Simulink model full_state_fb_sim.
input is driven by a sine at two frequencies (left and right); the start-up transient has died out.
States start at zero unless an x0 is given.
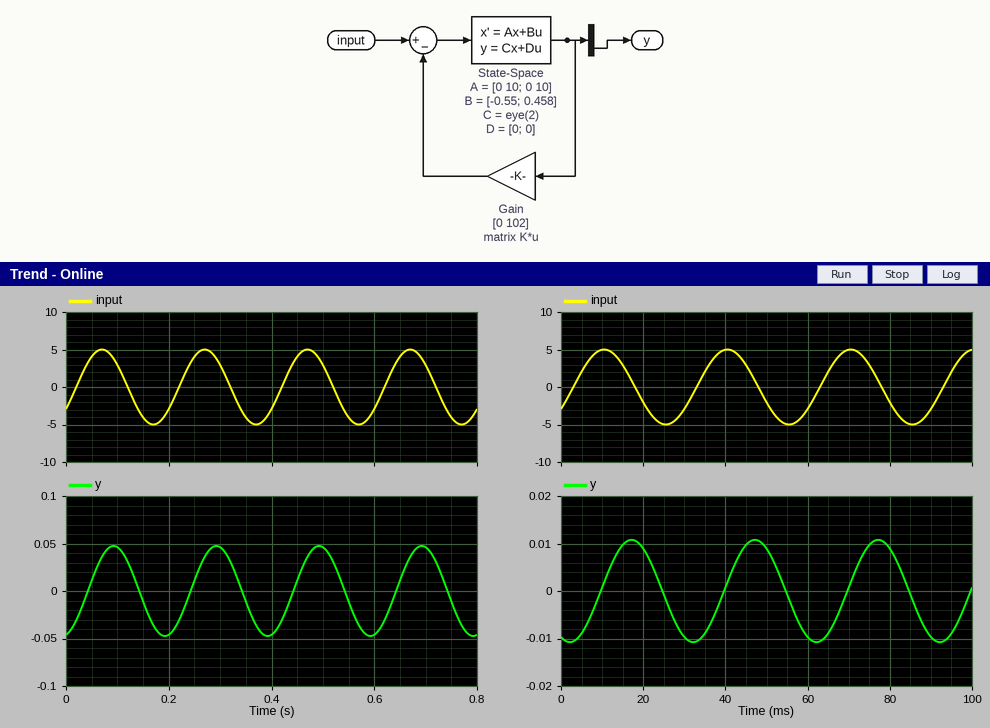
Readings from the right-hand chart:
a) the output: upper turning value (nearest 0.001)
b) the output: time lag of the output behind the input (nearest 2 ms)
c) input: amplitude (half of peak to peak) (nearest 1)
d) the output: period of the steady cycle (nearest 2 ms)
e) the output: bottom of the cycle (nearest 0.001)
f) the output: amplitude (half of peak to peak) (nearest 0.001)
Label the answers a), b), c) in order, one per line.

a) 0.011
b) 6 ms
c) 5
d) 30 ms
e) -0.011
f) 0.011
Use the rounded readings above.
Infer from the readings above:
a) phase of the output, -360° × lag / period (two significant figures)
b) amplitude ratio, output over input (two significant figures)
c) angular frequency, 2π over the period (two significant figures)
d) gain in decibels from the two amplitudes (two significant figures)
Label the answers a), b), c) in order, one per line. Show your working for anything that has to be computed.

a) -360 × 6 / 30 = -72°
b) 0.011 / 5 = 0.0022
c) 2π / 30 = 0.21 rad/ms
d) 20 log10(0.011 / 5) = -53 dB
